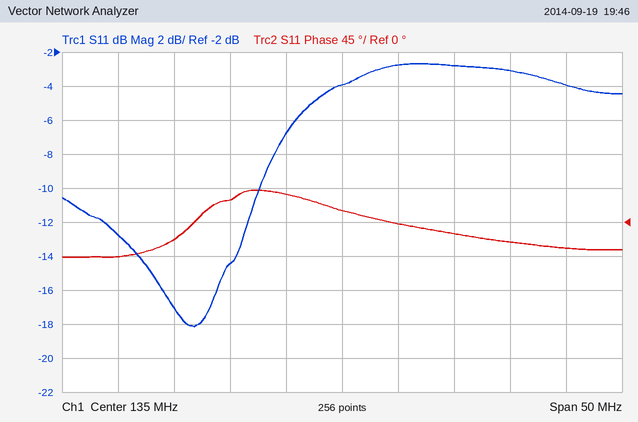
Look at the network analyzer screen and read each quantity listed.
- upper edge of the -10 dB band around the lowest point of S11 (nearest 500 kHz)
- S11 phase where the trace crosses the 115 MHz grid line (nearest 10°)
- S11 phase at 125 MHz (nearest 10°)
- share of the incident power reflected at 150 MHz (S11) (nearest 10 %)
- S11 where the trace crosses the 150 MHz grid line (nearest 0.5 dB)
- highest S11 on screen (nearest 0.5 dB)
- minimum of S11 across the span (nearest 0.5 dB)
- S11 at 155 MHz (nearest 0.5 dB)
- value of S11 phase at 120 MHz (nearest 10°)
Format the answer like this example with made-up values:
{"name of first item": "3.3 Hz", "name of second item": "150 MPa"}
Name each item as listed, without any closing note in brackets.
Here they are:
{"upper edge of the -10 dB band around the lowest point of S11": "127.5 MHz", "S11 phase where the trace crosses the 115 MHz grid line": "-50°", "S11 phase at 125 MHz": "30°", "share of the incident power reflected at 150 MHz (S11)": "50 %", "S11 where the trace crosses the 150 MHz grid line": "-3.0 dB", "highest S11 on screen": "-2.5 dB", "minimum of S11 across the span": "-18.0 dB", "S11 at 155 MHz": "-4.0 dB", "value of S11 phase at 120 MHz": "-20°"}
